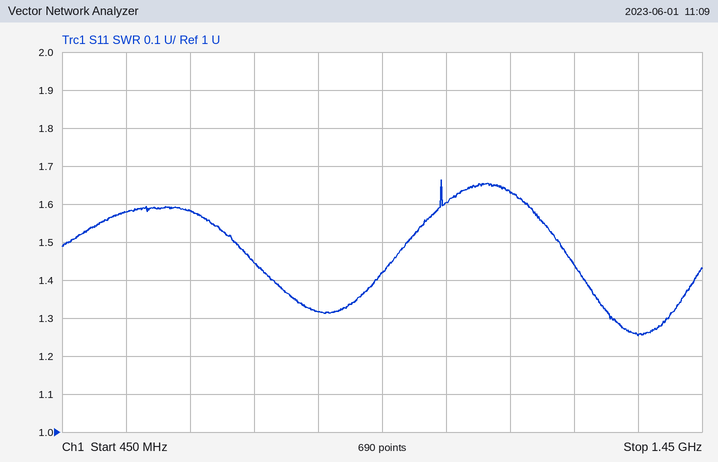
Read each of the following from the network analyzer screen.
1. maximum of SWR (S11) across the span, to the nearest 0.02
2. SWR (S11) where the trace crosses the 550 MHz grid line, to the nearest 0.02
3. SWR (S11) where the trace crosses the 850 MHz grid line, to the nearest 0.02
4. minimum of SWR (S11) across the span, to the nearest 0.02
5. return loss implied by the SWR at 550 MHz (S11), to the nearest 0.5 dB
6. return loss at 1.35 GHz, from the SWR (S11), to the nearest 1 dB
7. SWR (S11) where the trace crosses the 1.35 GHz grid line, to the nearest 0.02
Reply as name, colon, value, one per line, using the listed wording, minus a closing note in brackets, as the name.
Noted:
maximum of SWR (S11) across the span, to the nearest 0.02: 1.66
SWR (S11) where the trace crosses the 550 MHz grid line, to the nearest 0.02: 1.58
SWR (S11) where the trace crosses the 850 MHz grid line, to the nearest 0.02: 1.32
minimum of SWR (S11) across the span, to the nearest 0.02: 1.26
return loss implied by the SWR at 550 MHz (S11), to the nearest 0.5 dB: 13.0 dB
return loss at 1.35 GHz, from the SWR (S11), to the nearest 1 dB: 19 dB
SWR (S11) where the trace crosses the 1.35 GHz grid line, to the nearest 0.02: 1.26
